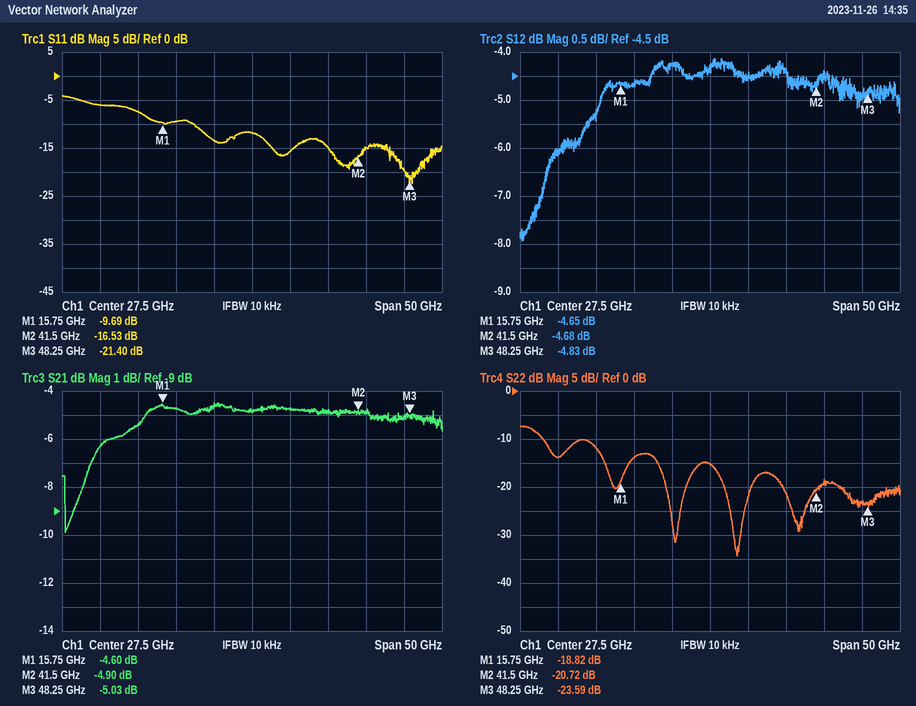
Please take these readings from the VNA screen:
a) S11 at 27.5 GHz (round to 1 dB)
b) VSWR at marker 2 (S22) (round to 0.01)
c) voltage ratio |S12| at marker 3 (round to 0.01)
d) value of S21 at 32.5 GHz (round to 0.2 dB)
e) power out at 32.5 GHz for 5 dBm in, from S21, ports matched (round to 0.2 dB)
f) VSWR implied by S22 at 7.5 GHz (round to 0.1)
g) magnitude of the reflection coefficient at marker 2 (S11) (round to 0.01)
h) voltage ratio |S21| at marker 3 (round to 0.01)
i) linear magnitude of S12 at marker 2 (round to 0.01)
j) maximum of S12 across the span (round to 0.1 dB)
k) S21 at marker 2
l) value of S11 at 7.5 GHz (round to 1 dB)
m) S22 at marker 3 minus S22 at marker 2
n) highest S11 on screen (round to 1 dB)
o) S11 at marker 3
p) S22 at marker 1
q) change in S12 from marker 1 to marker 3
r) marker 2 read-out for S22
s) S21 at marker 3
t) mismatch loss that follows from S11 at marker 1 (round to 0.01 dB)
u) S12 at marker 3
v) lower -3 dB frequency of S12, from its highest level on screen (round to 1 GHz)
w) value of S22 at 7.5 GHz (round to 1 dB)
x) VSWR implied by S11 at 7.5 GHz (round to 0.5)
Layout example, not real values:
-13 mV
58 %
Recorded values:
-12 dB
1.20
0.57
-4.8 dB
0.2 dBm
1.5
0.15
0.56
0.58
-4.1 dB
-4.90 dB
-6 dB
-2.87 dB
-4 dB
-21.40 dB
-18.82 dB
-0.18 dB
-20.72 dB
-5.03 dB
0.49 dB
-4.83 dB
5 GHz
-14 dB
3.0
